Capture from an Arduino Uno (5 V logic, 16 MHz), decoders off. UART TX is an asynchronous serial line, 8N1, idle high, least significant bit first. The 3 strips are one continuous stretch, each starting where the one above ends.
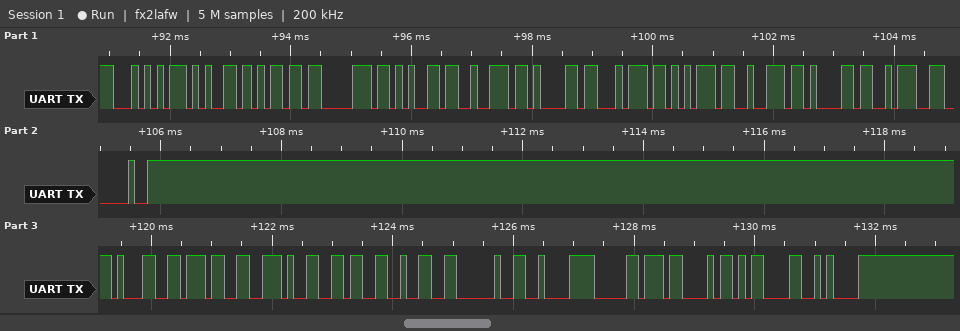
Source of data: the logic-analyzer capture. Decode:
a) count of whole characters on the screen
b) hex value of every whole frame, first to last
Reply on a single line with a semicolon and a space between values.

24; 0x54 0x65 0x6D 0x70 0x65 0x72 0x61 0x74 0x75 0x72 0x61 0x3A 0x20 0x31 0x37 0x2E 0x36 0x32 0x20 0xC2 0xB0 0x43 0x0D 0x0A
